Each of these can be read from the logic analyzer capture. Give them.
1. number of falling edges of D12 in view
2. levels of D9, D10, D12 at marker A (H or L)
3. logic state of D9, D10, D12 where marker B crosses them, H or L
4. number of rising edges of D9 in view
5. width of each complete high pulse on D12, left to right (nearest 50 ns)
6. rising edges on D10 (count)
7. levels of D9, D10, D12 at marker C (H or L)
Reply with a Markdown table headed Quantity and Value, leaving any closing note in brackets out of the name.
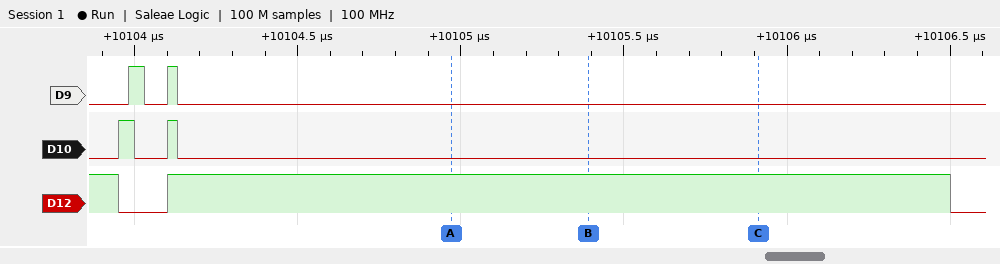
| Quantity | Value |
|---|---|
| number of falling edges of D12 in view | 2 |
| levels of D9, D10, D12 at marker A | D9=L, D10=L, D12=H |
| logic state of D9, D10, D12 where marker B crosses them, H or L | D9=L, D10=L, D12=H |
| number of rising edges of D9 in view | 2 |
| width of each complete high pulse on D12, left to right | 2400 ns |
| rising edges on D10 | 2 |
| levels of D9, D10, D12 at marker C | D9=L, D10=L, D12=H |
